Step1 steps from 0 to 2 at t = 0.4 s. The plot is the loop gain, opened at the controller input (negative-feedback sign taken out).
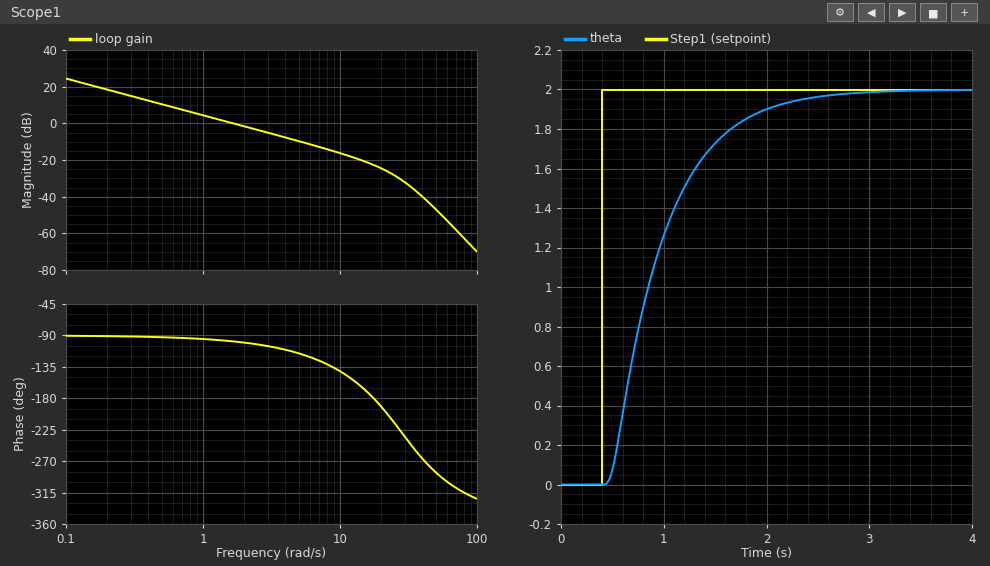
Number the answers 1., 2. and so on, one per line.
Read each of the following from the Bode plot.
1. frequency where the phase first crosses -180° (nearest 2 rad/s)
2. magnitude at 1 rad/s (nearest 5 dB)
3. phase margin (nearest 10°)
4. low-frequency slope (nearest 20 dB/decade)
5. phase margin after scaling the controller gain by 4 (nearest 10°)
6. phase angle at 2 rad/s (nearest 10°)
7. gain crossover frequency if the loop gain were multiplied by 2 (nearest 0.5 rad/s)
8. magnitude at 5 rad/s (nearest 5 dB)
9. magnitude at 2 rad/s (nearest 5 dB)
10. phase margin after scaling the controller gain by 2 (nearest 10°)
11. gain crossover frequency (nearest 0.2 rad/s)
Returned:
1. 18 rad/s
2. 5 dB
3. 80°
4. -20 dB/decade
5. 60°
6. -100°
7. 3.5 rad/s
8. -10 dB
9. 0 dB
10. 70°
11. 1.6 rad/s
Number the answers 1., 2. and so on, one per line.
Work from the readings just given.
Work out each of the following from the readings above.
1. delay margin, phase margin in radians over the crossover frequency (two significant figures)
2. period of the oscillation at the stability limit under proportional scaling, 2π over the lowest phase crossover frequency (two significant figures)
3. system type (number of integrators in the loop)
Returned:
1. 0.87 s
2. 0.35 s
3. 1
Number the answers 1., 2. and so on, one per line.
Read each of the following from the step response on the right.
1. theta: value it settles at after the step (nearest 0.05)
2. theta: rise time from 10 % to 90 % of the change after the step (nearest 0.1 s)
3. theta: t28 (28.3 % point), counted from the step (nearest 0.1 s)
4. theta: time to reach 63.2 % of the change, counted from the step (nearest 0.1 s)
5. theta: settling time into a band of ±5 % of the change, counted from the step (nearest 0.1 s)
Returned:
1. 2.00
2. 1.1 s
3. 0.3 s
4. 0.6 s
5. 1.6 s
